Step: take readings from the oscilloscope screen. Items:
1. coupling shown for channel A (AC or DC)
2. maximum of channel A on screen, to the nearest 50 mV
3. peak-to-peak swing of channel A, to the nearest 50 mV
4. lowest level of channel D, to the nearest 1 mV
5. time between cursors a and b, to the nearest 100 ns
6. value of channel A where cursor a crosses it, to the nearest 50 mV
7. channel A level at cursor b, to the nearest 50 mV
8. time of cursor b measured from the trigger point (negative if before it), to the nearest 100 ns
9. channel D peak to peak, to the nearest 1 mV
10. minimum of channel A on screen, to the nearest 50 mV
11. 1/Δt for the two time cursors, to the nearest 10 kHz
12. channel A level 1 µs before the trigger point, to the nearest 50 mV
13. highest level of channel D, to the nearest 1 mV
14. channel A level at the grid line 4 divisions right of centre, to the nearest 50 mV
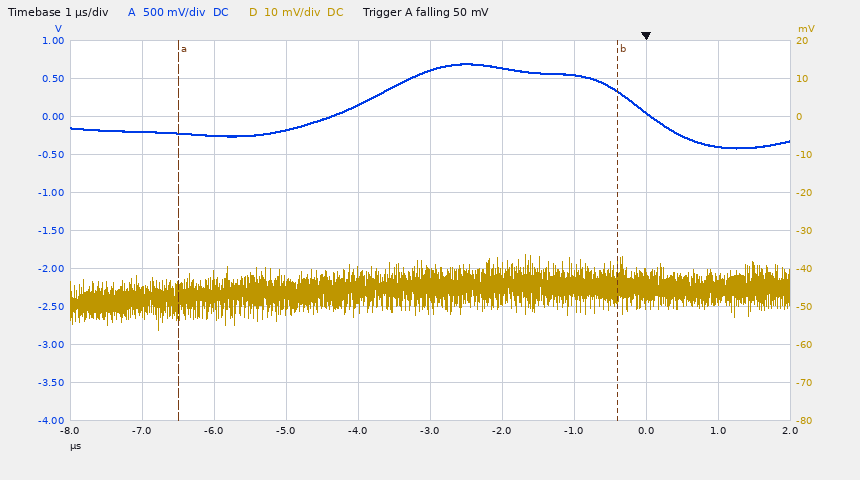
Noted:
DC
700 mV
1.10 V
-56 mV
6.1 µs
-200 mV
350 mV
-400 ns
20 mV
-400 mV
160 kHz
550 mV
-36 mV
-400 mV
